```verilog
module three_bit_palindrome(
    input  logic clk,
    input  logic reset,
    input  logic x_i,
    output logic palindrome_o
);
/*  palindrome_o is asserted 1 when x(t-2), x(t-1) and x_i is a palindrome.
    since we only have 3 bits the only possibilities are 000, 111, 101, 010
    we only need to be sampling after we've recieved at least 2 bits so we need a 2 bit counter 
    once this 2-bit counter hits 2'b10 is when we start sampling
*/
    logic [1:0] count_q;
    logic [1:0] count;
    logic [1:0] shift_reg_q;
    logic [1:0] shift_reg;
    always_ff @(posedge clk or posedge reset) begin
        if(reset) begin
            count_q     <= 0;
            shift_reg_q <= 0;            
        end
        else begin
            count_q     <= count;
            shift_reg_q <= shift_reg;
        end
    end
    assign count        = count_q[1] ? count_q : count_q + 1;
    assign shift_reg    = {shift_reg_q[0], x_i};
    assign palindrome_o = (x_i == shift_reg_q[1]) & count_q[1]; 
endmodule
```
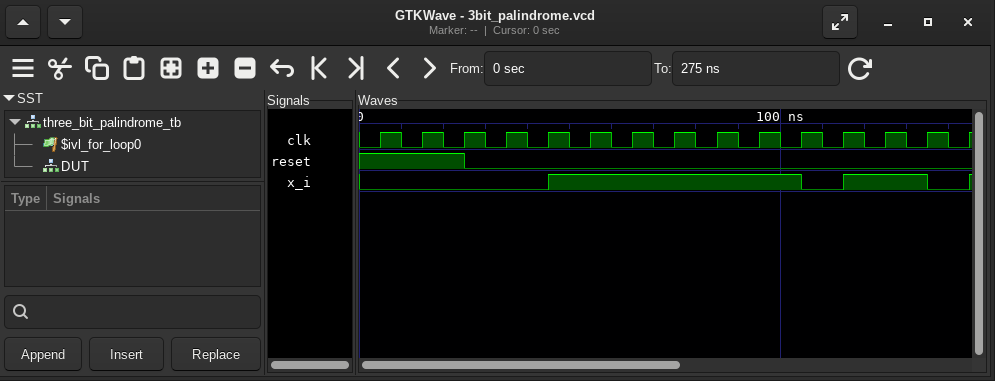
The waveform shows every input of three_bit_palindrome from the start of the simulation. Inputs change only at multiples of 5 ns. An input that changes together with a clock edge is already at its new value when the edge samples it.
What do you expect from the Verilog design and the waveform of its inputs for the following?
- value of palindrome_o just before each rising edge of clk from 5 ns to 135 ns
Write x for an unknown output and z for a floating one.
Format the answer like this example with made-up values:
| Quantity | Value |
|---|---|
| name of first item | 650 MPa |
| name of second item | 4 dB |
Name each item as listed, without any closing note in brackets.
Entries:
| Quantity | Value |
|---|---|
| value of palindrome_o just before each rising edge of clk from 5 ns to 135 ns | 0 0 0 0 1 0 1 1 1 1 1 0 0 1 |
